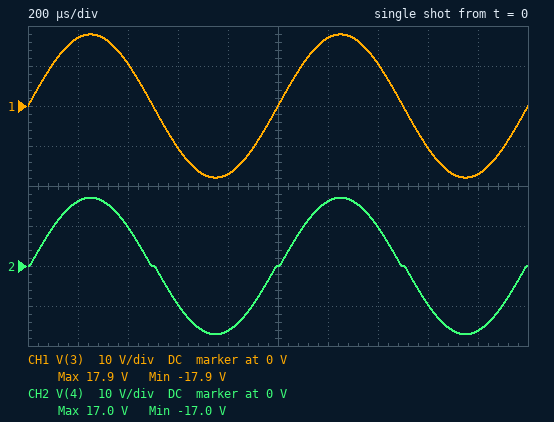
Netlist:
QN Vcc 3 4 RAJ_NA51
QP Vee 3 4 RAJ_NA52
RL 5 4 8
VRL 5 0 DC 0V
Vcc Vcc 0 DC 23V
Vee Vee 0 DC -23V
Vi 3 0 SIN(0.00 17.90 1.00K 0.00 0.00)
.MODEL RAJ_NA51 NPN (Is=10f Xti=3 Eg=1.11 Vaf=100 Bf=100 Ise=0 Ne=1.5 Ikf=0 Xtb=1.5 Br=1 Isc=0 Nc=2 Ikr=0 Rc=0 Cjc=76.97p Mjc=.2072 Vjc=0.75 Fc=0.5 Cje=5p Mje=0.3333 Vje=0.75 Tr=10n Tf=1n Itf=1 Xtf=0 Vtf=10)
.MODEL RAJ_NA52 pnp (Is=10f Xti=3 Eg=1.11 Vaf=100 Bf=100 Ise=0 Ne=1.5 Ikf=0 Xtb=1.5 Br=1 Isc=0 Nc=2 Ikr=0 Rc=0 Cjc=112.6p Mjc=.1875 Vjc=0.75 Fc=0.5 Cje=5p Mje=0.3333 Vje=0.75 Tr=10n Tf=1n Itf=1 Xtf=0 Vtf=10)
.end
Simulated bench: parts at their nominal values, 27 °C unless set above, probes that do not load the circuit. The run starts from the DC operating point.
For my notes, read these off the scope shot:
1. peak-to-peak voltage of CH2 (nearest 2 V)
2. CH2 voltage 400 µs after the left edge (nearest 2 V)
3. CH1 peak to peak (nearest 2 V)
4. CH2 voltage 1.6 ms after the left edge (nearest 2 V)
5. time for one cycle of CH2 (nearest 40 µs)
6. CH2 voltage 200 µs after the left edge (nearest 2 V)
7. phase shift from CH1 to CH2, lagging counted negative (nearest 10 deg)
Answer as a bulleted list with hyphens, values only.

- 34 V
- 10 V
- 36 V
- -10 V
- 1.00 ms
- 16 V
- 0 deg
